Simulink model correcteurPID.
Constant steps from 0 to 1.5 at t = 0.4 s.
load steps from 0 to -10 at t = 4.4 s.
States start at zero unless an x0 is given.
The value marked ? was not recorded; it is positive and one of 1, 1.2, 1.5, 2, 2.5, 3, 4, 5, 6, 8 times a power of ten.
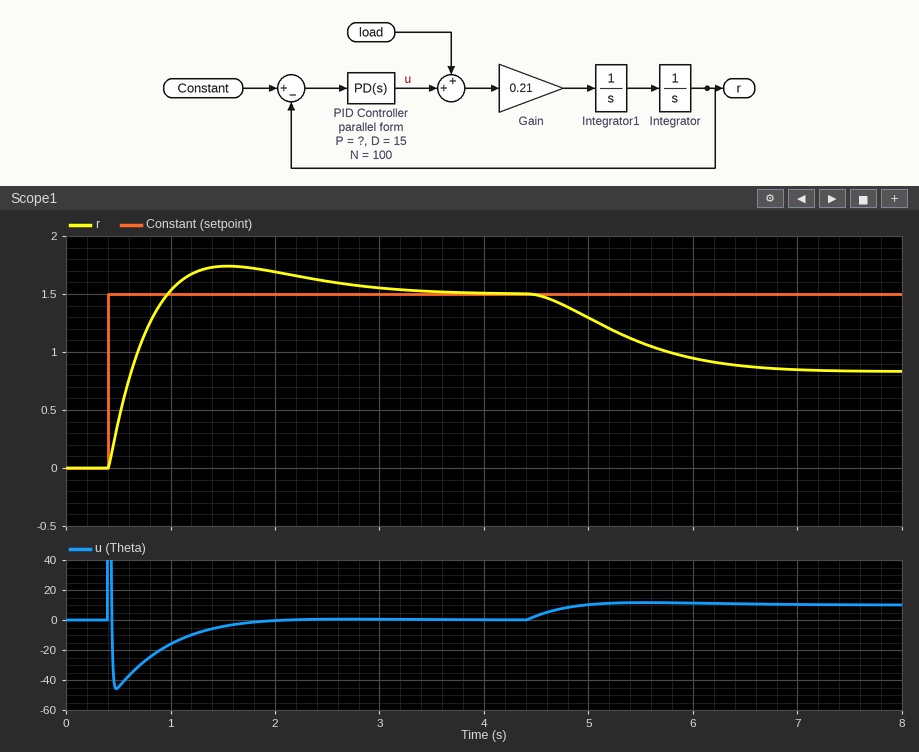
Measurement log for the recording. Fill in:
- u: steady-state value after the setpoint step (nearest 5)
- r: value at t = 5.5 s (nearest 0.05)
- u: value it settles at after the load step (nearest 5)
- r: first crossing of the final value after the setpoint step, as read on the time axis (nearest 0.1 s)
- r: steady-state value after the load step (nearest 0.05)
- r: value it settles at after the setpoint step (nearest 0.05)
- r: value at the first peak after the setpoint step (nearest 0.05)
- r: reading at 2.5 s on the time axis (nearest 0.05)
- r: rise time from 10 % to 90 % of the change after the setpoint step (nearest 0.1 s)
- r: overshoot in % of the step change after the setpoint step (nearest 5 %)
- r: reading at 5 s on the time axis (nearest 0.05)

0
1.10
10
1.0 s
0.85
1.50
1.75
1.60
0.4 s
15 %
1.30
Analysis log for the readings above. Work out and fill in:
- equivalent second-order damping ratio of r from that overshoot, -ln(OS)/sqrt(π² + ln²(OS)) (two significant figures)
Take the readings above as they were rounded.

0.52
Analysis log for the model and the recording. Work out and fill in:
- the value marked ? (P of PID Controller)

15
